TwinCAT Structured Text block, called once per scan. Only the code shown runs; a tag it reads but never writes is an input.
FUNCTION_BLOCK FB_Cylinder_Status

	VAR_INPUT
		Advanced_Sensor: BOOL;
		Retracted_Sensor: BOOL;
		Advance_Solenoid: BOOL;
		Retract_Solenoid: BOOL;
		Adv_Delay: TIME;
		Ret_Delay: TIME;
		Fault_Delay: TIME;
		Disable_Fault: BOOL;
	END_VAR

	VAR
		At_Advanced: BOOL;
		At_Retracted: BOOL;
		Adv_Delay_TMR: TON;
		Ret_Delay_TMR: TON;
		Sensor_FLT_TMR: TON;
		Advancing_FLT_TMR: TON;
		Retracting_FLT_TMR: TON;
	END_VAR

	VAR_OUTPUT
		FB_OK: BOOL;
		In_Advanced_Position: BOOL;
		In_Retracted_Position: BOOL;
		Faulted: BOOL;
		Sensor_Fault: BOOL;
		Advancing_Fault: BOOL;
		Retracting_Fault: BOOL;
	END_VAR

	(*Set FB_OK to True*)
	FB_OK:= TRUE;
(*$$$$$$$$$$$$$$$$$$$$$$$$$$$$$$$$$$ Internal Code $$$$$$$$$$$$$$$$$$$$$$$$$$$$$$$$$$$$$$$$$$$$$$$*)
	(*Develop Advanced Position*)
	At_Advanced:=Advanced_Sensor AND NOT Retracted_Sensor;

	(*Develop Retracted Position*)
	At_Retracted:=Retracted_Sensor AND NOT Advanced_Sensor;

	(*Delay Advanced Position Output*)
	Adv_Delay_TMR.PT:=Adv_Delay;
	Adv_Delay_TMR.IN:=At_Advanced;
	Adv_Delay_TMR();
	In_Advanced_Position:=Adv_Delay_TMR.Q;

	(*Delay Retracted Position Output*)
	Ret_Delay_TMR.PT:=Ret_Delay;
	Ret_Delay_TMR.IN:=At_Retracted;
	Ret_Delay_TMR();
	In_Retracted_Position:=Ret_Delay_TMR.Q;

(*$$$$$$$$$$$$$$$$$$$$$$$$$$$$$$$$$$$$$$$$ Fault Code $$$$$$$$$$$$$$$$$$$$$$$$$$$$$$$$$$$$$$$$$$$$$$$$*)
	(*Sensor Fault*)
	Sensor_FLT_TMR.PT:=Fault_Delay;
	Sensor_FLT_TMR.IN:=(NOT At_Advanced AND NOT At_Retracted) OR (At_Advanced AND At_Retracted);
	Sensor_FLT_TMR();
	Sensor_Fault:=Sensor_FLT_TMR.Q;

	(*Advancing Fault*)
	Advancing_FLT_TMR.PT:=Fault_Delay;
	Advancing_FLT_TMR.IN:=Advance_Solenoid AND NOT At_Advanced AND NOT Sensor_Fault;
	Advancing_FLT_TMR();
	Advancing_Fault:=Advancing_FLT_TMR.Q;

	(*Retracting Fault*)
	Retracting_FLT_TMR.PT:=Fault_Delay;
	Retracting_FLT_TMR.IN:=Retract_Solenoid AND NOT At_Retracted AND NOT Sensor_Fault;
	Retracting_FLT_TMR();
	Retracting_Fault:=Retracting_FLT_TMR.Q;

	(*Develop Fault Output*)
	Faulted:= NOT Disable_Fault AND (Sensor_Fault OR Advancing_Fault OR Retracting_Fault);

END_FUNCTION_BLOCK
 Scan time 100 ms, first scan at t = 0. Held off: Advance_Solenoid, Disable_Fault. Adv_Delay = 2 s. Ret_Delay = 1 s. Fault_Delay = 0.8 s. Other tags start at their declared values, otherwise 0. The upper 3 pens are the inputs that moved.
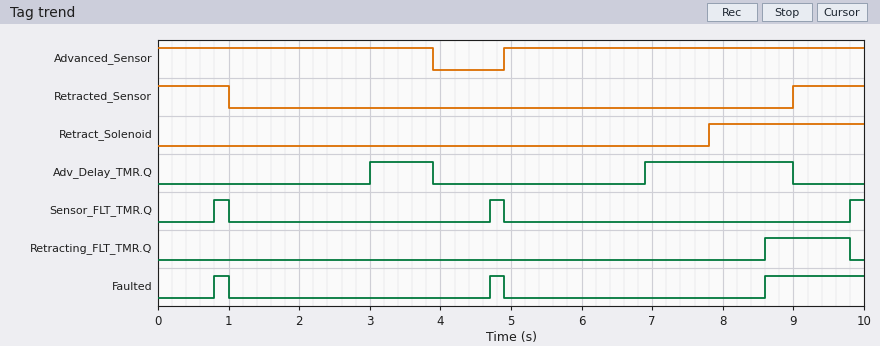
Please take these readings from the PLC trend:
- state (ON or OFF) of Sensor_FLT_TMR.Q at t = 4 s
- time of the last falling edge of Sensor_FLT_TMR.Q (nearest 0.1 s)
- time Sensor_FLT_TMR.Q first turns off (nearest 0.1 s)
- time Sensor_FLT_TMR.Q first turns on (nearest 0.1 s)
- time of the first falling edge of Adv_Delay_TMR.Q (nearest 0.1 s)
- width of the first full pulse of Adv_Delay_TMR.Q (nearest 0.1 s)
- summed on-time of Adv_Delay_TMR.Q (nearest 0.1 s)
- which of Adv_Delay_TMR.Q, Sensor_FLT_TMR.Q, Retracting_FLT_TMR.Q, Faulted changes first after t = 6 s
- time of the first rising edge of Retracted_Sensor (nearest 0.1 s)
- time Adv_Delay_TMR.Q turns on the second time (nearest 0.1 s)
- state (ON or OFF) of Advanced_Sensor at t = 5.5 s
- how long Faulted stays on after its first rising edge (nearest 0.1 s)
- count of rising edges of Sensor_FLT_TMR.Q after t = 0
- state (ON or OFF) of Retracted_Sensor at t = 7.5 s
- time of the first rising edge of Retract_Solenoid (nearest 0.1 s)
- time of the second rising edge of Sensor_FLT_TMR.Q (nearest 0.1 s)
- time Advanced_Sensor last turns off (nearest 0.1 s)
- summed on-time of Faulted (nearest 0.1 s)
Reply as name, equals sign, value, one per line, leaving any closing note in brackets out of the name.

state (ON or OFF) of Sensor_FLT_TMR.Q at t = 4 s = OFF
time of the last falling edge of Sensor_FLT_TMR.Q = 4.9 s
time Sensor_FLT_TMR.Q first turns off = 1.0 s
time Sensor_FLT_TMR.Q first turns on = 0.8 s
time of the first falling edge of Adv_Delay_TMR.Q = 3.9 s
width of the first full pulse of Adv_Delay_TMR.Q = 0.9 s
summed on-time of Adv_Delay_TMR.Q = 3.0 s
which of Adv_Delay_TMR.Q, Sensor_FLT_TMR.Q, Retracting_FLT_TMR.Q, Faulted changes first after t = 6 s = Adv_Delay_TMR.Q
time of the first rising edge of Retracted_Sensor = 9.0 s
time Adv_Delay_TMR.Q turns on the second time = 6.9 s
state (ON or OFF) of Advanced_Sensor at t = 5.5 s = ON
how long Faulted stays on after its first rising edge = 0.2 s
count of rising edges of Sensor_FLT_TMR.Q after t = 0 = 3
state (ON or OFF) of Retracted_Sensor at t = 7.5 s = OFF
time of the first rising edge of Retract_Solenoid = 7.8 s
time of the second rising edge of Sensor_FLT_TMR.Q = 4.7 s
time Advanced_Sensor last turns off = 3.9 s
summed on-time of Faulted = 1.8 s
